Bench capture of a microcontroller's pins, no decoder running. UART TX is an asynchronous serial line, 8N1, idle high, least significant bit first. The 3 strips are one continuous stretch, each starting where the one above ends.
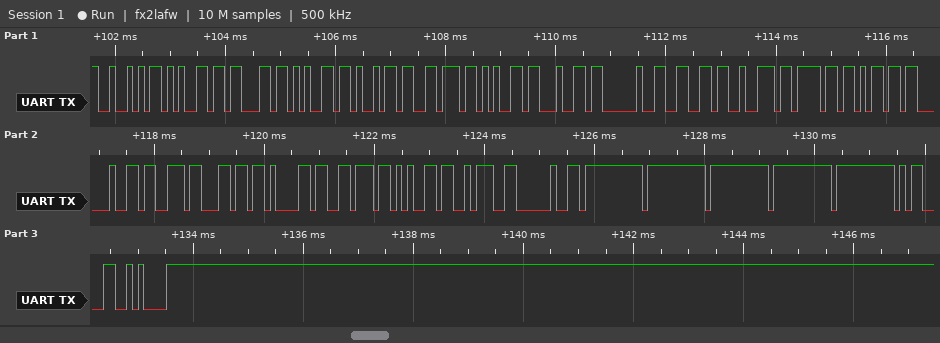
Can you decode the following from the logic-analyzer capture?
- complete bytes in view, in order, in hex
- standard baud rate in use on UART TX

52 65 63 65 69 76 65 64 20 66 72 6F 6D 20 73 6C 61 76 65 3A 20 FF FF FF FF FF 0D 0A
9600 baud
